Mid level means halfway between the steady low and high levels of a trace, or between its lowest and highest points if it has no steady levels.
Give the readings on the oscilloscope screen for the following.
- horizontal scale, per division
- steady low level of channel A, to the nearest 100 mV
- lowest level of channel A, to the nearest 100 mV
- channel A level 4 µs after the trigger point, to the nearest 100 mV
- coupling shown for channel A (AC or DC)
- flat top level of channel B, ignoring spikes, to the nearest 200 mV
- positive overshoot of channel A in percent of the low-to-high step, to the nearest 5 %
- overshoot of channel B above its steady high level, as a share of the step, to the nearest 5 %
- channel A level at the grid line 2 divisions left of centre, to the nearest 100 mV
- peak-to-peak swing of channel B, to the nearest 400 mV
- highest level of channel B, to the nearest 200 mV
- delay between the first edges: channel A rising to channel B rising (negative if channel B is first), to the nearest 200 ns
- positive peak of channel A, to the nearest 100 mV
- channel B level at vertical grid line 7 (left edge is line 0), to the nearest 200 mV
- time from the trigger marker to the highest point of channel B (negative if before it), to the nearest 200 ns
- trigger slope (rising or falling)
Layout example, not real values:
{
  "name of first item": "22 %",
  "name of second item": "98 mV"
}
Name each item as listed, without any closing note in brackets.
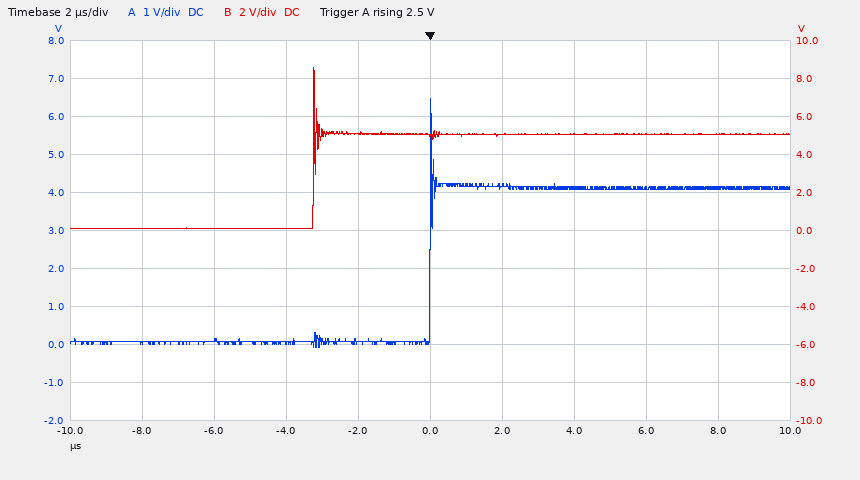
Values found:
{
  "horizontal scale, per division": "2 µs",
  "steady low level of channel A, to the nearest 100 mV": "100 mV",
  "lowest level of channel A, to the nearest 100 mV": "-100 mV",
  "channel A level 4 µs after the trigger point, to the nearest 100 mV": "4.1 V",
  "coupling shown for channel A": "DC",
  "flat top level of channel B, ignoring spikes, to the nearest 200 mV": "5.0 V",
  "positive overshoot of channel A in percent of the low-to-high step, to the nearest 5 %": "60 %",
  "overshoot of channel B above its steady high level, as a share of the step, to the nearest 5 %": "70 %",
  "channel A level at the grid line 2 divisions left of centre, to the nearest 100 mV": "0.0 V",
  "peak-to-peak swing of channel B, to the nearest 400 mV": "8.4 V",
  "highest level of channel B, to the nearest 200 mV": "8.6 V",
  "delay between the first edges: channel A rising to channel B rising (negative if channel B is first), to the nearest 200 ns": "-3.2 µs",
  "positive peak of channel A, to the nearest 100 mV": "6.5 V",
  "channel B level at vertical grid line 7 (left edge is line 0), to the nearest 200 mV": "5.0 V",
  "time from the trigger marker to the highest point of channel B (negative if before it), to the nearest 200 ns": "-3.2 µs",
  "trigger slope": "rising"
}
